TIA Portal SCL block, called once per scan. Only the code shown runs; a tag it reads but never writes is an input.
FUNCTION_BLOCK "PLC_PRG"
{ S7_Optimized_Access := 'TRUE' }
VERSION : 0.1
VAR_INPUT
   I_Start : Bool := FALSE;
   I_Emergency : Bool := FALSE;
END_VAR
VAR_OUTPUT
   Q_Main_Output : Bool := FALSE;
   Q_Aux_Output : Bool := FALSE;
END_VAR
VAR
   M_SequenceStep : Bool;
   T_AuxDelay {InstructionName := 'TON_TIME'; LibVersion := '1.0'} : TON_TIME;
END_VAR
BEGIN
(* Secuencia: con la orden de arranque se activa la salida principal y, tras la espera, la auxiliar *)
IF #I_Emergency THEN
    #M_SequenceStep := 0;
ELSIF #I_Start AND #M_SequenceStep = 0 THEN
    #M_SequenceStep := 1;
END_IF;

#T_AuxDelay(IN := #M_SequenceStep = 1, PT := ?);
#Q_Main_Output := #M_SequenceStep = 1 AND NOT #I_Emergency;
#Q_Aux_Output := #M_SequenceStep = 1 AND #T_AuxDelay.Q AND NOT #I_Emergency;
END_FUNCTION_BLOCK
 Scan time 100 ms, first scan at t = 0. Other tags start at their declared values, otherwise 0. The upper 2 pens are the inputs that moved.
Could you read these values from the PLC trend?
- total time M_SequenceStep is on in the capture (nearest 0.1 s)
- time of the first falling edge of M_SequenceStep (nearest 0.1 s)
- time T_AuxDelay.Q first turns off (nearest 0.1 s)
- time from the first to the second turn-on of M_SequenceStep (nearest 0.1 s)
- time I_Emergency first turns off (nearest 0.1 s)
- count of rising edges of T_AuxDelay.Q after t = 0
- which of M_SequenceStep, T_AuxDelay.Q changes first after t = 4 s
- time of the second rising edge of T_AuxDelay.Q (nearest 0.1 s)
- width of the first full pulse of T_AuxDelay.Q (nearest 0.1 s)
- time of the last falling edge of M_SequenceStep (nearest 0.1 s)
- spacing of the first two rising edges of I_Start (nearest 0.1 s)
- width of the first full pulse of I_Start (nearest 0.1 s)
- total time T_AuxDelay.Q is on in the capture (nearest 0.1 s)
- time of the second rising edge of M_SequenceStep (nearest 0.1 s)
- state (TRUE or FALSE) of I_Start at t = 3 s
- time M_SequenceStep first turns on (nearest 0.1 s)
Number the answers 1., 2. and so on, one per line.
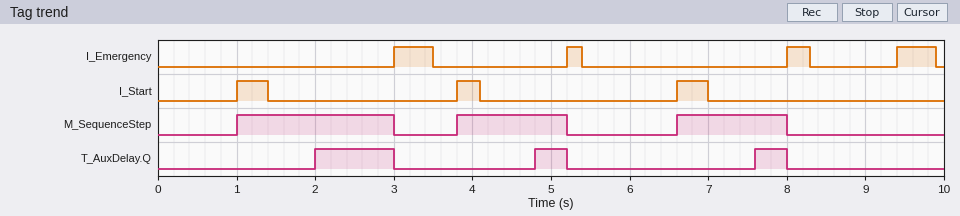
1. 4.8 s
2. 3.0 s
3. 3.0 s
4. 2.8 s
5. 3.5 s
6. 3
7. T_AuxDelay.Q
8. 4.8 s
9. 1.0 s
10. 8.0 s
11. 2.8 s
12. 0.4 s
13. 1.8 s
14. 3.8 s
15. FALSE
16. 1.0 s
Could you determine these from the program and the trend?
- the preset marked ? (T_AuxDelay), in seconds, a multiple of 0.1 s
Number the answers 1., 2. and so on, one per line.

1. 1.0 s
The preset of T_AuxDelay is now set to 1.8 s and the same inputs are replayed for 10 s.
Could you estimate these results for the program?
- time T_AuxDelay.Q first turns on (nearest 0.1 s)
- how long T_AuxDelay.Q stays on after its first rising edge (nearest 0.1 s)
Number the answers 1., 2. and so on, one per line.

1. 2.8 s
2. 0.2 s
